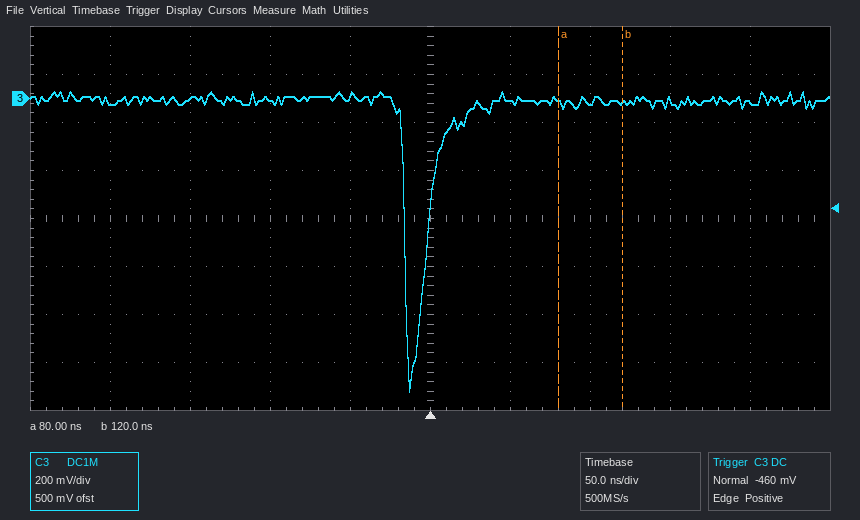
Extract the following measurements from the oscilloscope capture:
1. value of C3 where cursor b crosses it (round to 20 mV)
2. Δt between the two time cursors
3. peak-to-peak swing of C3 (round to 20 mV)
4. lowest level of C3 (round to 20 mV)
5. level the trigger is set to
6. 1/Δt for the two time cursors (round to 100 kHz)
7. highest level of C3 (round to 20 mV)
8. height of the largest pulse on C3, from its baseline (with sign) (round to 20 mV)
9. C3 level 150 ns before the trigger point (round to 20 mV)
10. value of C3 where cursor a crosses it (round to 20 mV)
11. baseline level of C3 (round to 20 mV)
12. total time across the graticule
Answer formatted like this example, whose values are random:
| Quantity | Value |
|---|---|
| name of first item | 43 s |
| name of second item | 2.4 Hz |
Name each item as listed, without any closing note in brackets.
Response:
| Quantity | Value |
|---|---|
| value of C3 where cursor b crosses it | -20 mV |
| Δt between the two time cursors | 40 ns |
| peak-to-peak swing of C3 | 1.24 V |
| lowest level of C3 | -1.22 V |
| level the trigger is set to | -460 mV |
| 1/Δt for the two time cursors | 25.0 MHz |
| highest level of C3 | 20 mV |
| height of the largest pulse on C3, from its baseline (with sign) | -1.22 V |
| C3 level 150 ns before the trigger point | 0 mV |
| value of C3 where cursor a crosses it | -20 mV |
| baseline level of C3 | 0 mV |
| total time across the graticule | 500 ns |
